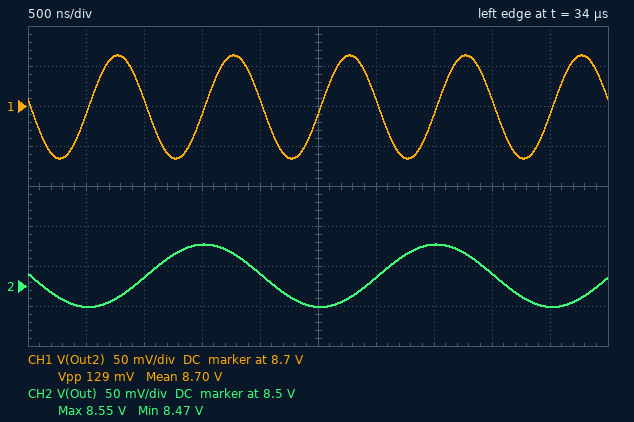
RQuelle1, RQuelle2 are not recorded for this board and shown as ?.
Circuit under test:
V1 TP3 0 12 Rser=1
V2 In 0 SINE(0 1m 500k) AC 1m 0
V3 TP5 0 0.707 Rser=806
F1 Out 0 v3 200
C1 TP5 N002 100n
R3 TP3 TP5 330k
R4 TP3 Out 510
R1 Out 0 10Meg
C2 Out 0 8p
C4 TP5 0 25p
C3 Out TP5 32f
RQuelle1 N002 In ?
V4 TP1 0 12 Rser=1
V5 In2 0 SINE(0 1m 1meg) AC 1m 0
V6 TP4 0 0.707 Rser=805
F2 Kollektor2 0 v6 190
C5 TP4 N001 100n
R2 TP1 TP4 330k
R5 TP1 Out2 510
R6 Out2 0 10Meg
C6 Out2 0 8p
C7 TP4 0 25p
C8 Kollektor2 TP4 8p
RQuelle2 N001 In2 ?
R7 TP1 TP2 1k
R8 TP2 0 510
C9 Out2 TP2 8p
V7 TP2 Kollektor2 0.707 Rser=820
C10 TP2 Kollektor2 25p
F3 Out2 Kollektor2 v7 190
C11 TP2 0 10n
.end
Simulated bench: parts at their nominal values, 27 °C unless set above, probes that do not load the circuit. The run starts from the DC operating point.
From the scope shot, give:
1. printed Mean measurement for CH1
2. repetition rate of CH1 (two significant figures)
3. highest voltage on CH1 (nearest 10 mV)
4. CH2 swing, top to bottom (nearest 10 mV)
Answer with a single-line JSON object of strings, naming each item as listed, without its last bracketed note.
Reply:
{"printed Mean measurement for CH1": "8.70 V", "repetition rate of CH1": "1.0 MHz", "highest voltage on CH1": "8.76 V", "CH2 swing, top to bottom": "80 mV"}
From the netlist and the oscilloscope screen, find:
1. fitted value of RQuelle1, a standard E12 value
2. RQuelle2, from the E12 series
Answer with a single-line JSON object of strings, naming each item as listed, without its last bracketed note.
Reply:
{"fitted value of RQuelle1, a standard E12 value": "1.8 kΩ", "RQuelle2, from the E12 series": "680 Ω"}
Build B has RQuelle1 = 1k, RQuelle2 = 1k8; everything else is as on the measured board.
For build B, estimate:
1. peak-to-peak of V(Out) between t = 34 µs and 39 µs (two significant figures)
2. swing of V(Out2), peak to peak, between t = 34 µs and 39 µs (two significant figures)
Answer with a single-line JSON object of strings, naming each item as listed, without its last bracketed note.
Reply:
{"peak-to-peak of V(Out) between t = 34 µs and 39 µs": "110 mV", "swing of V(Out2), peak to peak, between t = 34 µs and 39 µs": "73 mV"}
